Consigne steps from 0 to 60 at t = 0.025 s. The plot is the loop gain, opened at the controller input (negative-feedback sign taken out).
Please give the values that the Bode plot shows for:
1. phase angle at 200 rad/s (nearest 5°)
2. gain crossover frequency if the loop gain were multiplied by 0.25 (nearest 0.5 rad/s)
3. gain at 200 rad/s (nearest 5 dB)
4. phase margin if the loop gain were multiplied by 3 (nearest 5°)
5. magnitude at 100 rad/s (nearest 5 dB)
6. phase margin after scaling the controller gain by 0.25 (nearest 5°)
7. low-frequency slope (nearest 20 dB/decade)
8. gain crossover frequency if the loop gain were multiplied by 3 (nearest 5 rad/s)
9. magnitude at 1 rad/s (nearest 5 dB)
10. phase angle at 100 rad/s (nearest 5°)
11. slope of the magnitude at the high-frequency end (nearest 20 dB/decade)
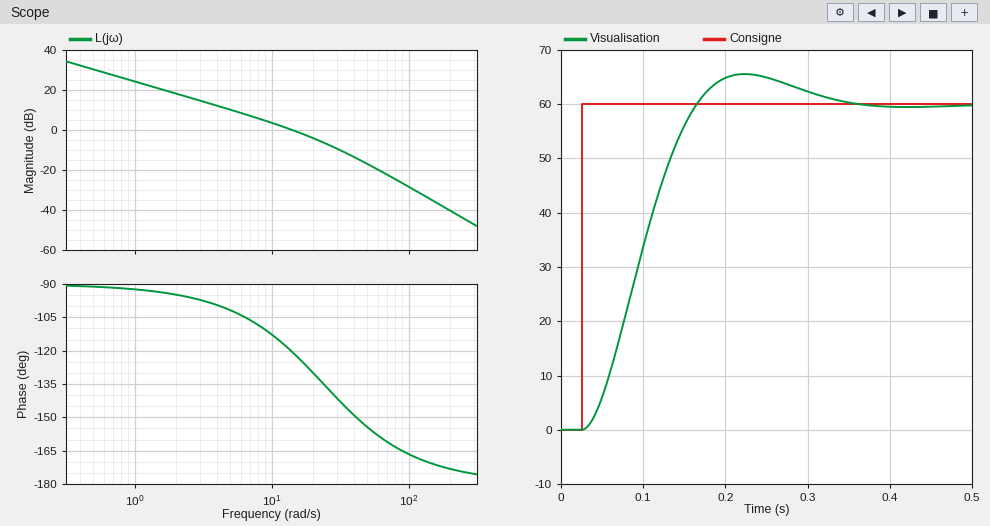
-175°
4.0 rad/s
-40 dB
40°
-30 dB
80°
-20 dB/decade
30 rad/s
25 dB
-165°
-40 dB/decade
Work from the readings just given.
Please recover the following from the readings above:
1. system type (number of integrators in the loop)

1
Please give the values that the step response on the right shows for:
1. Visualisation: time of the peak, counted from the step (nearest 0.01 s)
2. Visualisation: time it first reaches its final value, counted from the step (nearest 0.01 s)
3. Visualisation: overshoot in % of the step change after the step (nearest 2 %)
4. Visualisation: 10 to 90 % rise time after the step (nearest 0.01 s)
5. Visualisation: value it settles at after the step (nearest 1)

0.20 s
0.14 s
10 %
0.09 s
60
